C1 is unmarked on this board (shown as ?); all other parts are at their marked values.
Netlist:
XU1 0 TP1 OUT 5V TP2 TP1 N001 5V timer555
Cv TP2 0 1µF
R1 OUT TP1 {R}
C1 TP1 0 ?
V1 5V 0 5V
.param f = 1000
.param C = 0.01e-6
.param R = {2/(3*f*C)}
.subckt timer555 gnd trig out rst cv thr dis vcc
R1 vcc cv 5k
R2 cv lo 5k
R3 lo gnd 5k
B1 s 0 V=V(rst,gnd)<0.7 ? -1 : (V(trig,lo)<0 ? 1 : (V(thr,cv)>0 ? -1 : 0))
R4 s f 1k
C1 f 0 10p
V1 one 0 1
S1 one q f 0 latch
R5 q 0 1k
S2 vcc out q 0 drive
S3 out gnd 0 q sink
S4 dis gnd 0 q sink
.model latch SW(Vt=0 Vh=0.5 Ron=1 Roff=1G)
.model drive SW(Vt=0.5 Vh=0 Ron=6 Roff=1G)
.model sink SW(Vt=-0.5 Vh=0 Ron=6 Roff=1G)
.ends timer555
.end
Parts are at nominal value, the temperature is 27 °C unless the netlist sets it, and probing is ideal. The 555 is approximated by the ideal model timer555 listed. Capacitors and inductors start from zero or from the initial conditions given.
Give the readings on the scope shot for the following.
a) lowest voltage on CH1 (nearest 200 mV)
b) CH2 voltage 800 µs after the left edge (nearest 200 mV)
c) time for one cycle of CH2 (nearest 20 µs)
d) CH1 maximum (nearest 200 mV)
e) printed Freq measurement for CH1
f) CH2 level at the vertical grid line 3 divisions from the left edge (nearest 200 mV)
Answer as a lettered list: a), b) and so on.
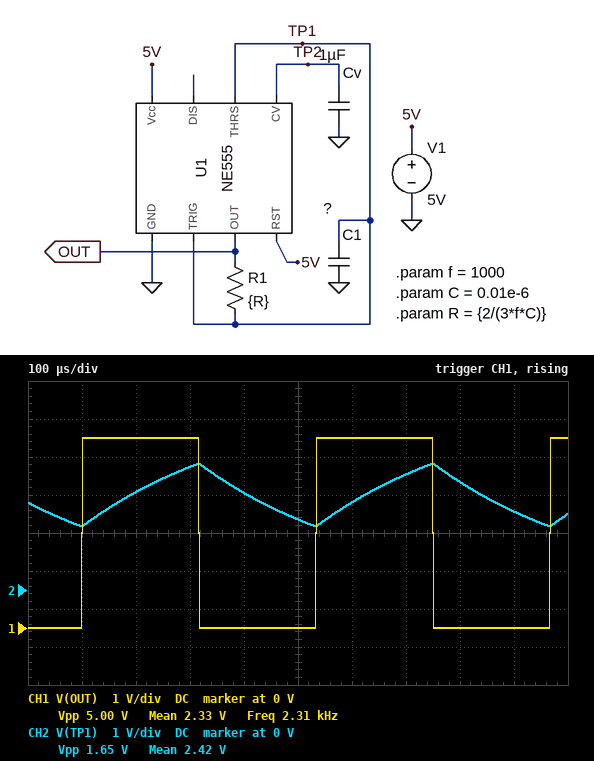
a) 0 V
b) 2.8 V
c) 440 µs
d) 5.0 V
e) 2.31 kHz
f) 3.2 V
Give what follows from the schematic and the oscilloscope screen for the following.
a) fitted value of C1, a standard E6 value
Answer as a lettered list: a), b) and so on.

a) 4.7 nF
